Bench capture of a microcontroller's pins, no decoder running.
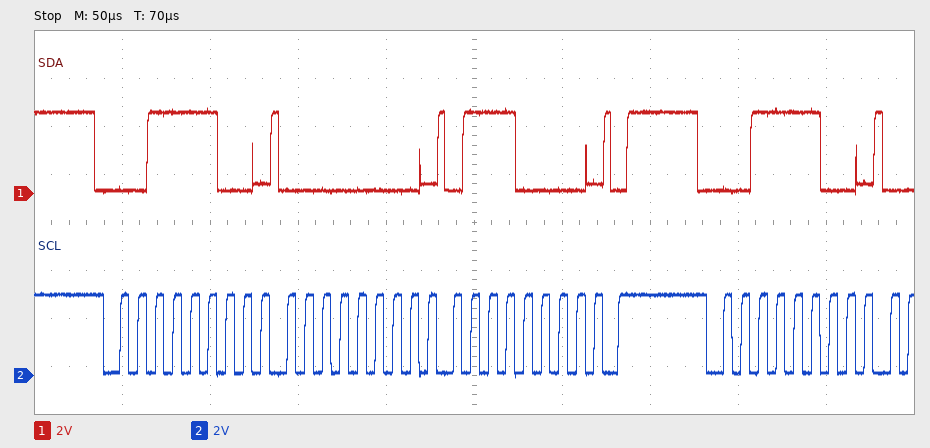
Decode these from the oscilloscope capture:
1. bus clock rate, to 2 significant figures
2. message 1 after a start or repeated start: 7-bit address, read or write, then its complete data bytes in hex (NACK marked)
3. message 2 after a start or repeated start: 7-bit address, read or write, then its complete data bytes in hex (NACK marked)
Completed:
100 kHz
0x1E write: 00 70
0x1E write
